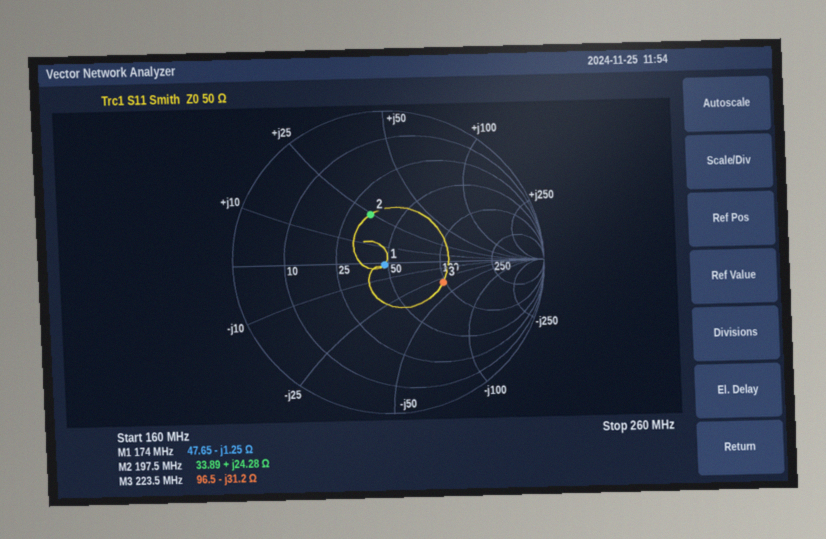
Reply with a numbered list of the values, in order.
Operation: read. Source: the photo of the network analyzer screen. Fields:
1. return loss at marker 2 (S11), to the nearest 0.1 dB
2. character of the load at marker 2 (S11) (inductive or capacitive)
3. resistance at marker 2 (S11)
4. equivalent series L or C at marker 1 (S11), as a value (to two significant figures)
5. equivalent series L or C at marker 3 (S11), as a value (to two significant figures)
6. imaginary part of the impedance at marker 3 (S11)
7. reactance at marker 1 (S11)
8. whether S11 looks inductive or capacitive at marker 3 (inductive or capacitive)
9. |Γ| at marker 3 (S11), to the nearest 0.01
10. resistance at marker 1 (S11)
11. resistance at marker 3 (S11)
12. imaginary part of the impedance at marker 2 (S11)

1. 9.5 dB
2. inductive
3. 33.89 Ω
4. 730 pF
5. 23 pF
6. -31.2 Ω
7. -1.25 Ω
8. capacitive
9. 0.37
10. 47.65 Ω
11. 96.5 Ω
12. +24.28 Ω
